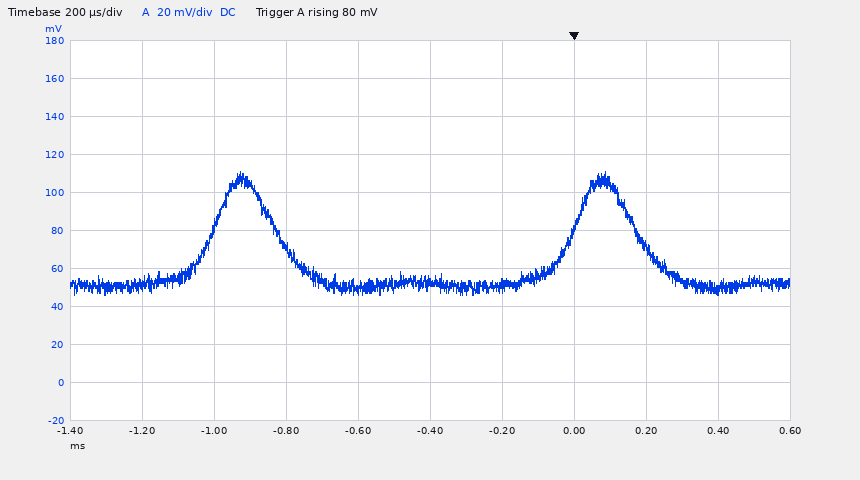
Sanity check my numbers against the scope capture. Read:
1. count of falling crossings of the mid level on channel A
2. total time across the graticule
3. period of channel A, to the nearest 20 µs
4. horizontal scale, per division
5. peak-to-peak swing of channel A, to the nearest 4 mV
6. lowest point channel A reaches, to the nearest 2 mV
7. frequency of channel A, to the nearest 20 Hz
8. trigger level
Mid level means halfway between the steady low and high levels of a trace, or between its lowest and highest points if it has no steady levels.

2
2 ms
1.00 ms
200 µs
64 mV
46 mV
1.00 kHz
80 mV
